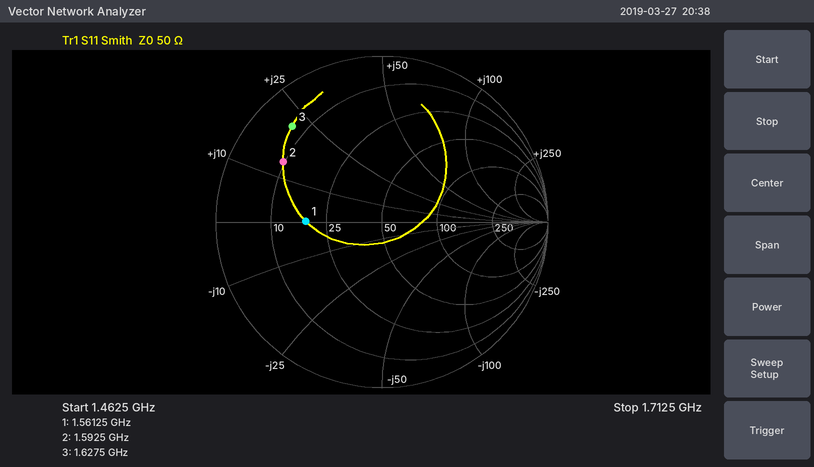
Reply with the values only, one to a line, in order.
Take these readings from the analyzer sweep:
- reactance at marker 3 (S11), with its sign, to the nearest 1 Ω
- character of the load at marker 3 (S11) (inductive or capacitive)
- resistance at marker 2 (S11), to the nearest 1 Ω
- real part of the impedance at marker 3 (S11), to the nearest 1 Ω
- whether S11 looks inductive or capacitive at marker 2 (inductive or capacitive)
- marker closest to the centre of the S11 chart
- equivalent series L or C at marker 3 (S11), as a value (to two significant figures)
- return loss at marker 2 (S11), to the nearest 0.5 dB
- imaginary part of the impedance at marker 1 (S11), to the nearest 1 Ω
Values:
+21 Ω
inductive
10 Ω
7 Ω
inductive
marker 1
2.1 nH
3.0 dB
0 Ω
